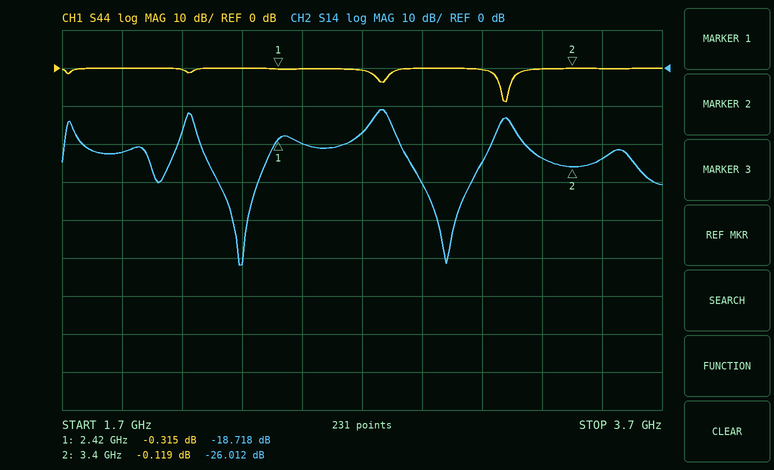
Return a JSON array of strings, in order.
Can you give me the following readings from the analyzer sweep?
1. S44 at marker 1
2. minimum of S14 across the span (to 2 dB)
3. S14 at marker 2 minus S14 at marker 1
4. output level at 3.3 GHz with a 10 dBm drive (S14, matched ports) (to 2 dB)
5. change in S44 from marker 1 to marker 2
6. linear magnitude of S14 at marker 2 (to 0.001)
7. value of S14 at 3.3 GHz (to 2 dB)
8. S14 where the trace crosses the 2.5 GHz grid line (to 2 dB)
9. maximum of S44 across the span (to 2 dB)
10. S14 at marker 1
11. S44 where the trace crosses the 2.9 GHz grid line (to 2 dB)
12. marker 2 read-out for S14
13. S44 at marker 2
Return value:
["-0.315 dB", "-52 dB", "-7.294 dB", "-14 dBm", "0.196 dB", "0.050", "-24 dB", "-20 dB", "0 dB", "-18.718 dB", "0 dB", "-26.012 dB", "-0.119 dB"]
